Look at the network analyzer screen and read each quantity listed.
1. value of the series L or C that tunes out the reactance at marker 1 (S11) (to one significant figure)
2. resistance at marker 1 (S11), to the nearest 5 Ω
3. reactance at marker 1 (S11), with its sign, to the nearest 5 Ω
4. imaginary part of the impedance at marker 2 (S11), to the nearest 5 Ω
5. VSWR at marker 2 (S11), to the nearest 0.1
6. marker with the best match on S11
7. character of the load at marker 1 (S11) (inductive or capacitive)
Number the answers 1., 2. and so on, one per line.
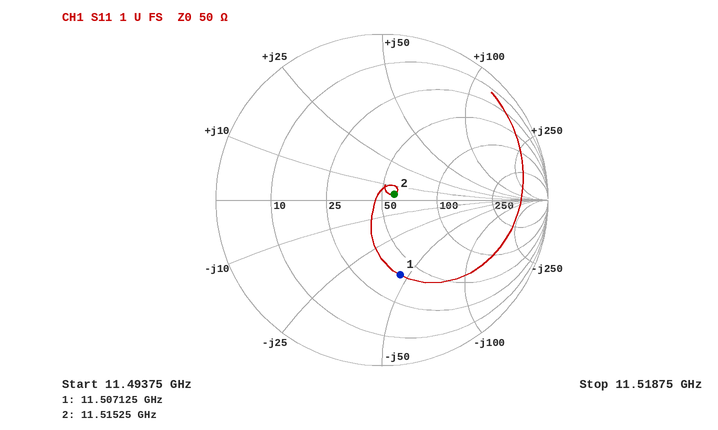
1. 600 pH
2. 40 Ω
3. -45 Ω
4. +5 Ω
5. 1.2
6. marker 2
7. capacitive
